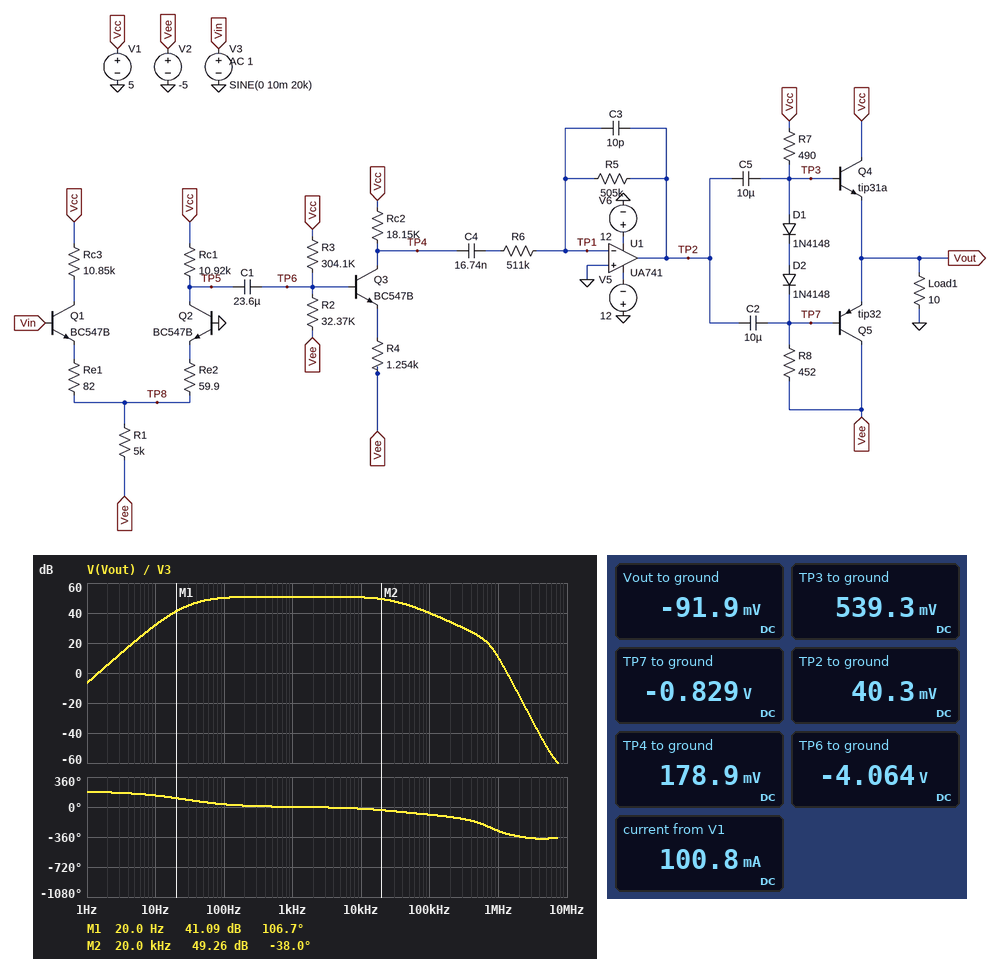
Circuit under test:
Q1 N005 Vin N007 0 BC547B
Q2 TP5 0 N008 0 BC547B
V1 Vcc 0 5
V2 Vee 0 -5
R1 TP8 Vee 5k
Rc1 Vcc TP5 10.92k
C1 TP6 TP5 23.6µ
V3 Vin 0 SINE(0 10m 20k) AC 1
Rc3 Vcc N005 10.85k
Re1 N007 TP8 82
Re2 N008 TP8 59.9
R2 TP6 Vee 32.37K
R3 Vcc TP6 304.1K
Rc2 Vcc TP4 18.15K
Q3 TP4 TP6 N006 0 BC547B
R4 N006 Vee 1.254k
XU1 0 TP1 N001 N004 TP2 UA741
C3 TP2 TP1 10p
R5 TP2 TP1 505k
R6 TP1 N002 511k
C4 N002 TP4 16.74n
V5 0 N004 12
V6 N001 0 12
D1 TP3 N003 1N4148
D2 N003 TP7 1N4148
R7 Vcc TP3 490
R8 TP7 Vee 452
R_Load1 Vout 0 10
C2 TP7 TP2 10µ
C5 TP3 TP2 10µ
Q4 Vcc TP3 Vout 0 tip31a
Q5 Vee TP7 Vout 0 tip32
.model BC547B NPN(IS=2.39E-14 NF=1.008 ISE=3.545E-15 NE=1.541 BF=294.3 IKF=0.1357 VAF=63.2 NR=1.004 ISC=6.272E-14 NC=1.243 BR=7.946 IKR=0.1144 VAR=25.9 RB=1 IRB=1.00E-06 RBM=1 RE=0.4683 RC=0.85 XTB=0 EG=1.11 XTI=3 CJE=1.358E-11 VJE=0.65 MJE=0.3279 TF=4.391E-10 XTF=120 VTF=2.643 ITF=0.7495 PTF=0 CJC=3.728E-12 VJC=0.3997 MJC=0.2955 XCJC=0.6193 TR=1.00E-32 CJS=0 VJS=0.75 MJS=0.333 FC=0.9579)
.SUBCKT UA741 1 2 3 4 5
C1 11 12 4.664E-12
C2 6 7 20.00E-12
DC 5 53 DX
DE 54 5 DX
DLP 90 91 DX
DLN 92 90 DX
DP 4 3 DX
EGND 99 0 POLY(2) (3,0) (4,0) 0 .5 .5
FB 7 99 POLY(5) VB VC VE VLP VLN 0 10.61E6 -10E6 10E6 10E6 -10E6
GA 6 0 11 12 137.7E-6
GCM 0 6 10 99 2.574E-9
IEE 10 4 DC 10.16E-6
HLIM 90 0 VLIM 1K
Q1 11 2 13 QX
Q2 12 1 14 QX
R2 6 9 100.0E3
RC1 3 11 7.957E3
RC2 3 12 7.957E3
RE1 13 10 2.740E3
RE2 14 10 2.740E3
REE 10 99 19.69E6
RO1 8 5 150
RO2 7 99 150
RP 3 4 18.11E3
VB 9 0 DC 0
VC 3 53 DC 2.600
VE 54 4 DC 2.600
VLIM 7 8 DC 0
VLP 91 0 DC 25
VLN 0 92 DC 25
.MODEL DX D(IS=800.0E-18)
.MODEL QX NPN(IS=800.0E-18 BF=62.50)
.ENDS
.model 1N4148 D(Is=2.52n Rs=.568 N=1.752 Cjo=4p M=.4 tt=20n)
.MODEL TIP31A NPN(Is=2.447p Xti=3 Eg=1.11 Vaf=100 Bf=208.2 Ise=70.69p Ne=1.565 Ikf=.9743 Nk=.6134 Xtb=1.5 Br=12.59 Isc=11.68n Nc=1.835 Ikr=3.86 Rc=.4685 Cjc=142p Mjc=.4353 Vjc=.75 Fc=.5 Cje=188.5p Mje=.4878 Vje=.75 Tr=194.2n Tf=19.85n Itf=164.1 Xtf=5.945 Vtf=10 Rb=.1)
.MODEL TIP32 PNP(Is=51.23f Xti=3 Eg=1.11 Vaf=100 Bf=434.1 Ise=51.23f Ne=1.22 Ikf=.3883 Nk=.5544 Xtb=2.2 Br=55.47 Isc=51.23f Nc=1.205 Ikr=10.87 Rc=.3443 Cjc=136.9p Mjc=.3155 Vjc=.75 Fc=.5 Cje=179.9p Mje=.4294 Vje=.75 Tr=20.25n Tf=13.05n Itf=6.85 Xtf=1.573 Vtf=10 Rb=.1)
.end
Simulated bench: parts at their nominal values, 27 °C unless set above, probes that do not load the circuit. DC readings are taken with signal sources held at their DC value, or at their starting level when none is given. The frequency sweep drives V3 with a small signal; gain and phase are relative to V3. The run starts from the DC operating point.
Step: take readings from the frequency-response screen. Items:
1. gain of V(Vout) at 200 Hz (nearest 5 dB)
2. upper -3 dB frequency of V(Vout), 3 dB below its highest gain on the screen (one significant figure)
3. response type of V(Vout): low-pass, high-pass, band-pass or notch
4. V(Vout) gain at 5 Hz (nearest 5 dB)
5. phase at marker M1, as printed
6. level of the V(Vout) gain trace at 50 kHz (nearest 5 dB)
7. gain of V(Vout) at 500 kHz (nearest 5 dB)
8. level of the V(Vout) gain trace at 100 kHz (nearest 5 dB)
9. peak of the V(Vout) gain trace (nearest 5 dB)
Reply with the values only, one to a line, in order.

50 dB
30 kHz
band-pass
20 dB
106.7 deg
45 dB
25 dB
40 dB
50 dB
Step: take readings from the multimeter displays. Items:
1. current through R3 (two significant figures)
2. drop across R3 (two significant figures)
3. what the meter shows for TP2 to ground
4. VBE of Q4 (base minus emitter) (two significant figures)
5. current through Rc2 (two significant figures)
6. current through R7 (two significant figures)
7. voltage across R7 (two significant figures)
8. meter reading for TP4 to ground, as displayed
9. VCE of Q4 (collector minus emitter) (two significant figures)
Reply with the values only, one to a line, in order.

30 µA
9.1 V
40.3 mV
630 mV
270 µA
9.1 mA
4.5 V
178.9 mV
5.1 V
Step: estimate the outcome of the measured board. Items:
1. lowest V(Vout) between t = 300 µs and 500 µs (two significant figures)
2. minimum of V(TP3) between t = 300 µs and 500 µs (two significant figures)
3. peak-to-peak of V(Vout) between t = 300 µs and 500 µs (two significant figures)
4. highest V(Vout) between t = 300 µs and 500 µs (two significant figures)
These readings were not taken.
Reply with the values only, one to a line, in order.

-2.8 V
-2.2 V
5.6 V
2.8 V
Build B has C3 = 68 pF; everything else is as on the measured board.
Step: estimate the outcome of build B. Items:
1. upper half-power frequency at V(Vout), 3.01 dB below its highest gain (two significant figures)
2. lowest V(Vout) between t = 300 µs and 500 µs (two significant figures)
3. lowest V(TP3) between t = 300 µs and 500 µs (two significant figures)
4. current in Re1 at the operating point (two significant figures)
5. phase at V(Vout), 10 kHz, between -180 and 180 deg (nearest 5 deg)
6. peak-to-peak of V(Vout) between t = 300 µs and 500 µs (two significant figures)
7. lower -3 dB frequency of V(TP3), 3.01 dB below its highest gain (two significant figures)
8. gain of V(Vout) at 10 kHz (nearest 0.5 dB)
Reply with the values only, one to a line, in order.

4.7 kHz
-820 mV
-200 mV
400 µA
-65 deg
1.6 V
47 Hz
43.5 dB
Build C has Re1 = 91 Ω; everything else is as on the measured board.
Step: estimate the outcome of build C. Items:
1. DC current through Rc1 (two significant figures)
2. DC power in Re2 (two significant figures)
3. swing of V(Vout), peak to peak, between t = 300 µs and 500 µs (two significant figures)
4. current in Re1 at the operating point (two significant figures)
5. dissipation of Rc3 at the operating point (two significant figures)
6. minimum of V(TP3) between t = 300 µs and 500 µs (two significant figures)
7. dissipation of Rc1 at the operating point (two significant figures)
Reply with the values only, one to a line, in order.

480 µA
14 µW
5.3 V
390 µA
1.6 mW
-2.0 V
2.5 mW
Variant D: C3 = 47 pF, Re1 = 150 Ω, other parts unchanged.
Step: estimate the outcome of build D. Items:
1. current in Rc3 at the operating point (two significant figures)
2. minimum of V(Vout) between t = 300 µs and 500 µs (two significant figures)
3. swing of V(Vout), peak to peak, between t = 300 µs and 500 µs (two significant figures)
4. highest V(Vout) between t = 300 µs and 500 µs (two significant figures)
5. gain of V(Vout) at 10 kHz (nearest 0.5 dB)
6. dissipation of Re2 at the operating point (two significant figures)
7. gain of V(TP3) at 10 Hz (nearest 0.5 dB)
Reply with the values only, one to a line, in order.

330 µA
-140 mV
180 mV
44 mV
23.0 dB
17 µW
9.5 dB
